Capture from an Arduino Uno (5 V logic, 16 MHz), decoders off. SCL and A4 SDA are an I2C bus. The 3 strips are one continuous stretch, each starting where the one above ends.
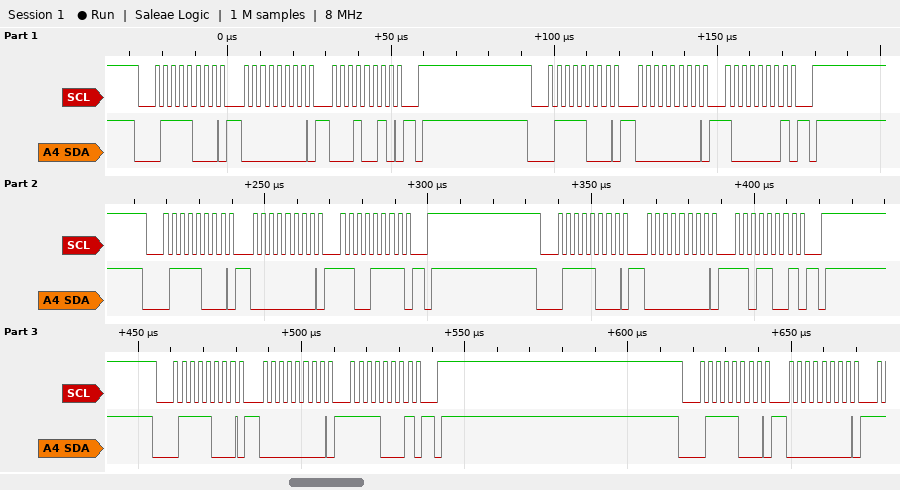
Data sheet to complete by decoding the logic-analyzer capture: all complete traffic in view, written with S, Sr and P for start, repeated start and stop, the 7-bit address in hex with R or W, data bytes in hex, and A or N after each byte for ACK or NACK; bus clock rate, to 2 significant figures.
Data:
S 3CW A 00 A 12 A P S 3CW A 00 A 81 A P S 3CW A 00 A CF A P S 3CW A 00 A D9 A P S 3CW A 00 A F1 A P S 3CW A 00 A
400 kHz
